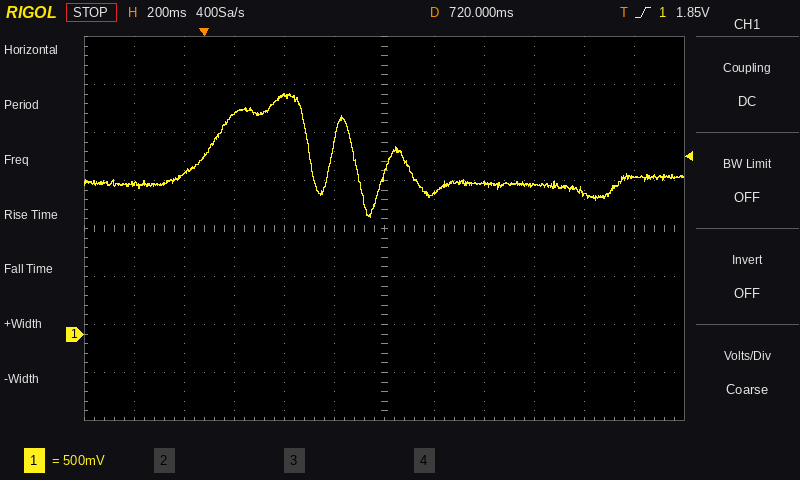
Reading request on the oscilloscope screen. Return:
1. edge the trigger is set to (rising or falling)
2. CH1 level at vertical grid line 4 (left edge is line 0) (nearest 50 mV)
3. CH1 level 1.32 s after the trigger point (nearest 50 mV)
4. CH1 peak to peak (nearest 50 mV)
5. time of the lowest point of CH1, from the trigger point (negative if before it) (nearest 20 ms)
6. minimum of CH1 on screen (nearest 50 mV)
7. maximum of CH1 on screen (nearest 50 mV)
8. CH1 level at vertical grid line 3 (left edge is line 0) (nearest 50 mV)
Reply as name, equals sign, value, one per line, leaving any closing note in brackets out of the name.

edge the trigger is set to = rising
CH1 level at vertical grid line 4 (left edge is line 0) = 2.50 V
CH1 level 1.32 s after the trigger point = 1.55 V
CH1 peak to peak = 1.30 V
time of the lowest point of CH1, from the trigger point (negative if before it) = +660 ms
minimum of CH1 on screen = 1.20 V
maximum of CH1 on screen = 2.50 V
CH1 level at vertical grid line 3 (left edge is line 0) = 2.30 V
